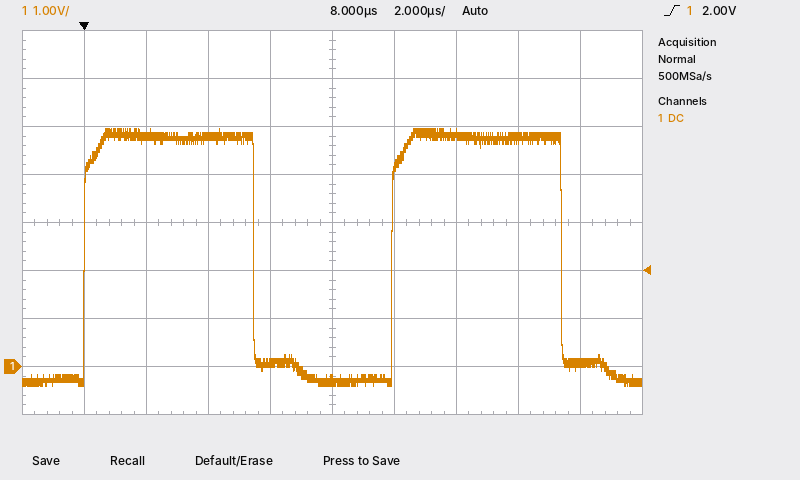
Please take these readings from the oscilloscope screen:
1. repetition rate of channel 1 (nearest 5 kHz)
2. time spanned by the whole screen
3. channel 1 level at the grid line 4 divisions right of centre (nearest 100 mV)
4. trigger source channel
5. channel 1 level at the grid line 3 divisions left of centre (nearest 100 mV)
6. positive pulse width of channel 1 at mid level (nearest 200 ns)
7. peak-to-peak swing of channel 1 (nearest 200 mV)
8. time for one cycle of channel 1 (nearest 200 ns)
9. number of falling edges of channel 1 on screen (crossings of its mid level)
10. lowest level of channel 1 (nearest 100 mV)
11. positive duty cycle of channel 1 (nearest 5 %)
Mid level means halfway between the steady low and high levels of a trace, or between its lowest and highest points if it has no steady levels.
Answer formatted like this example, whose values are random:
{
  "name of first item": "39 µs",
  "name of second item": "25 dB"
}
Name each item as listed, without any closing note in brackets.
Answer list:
{
  "repetition rate of channel 1": "100 kHz",
  "time spanned by the whole screen": "20 µs",
  "channel 1 level at the grid line 4 divisions right of centre": "100 mV",
  "trigger source channel": "channel 1",
  "channel 1 level at the grid line 3 divisions left of centre": "4.8 V",
  "positive pulse width of channel 1 at mid level": "5.4 µs",
  "peak-to-peak swing of channel 1": "5.4 V",
  "time for one cycle of channel 1": "10.0 µs",
  "number of falling edges of channel 1 on screen": "2",
  "lowest level of channel 1": "-400 mV",
  "positive duty cycle of channel 1": "55 %"
}
